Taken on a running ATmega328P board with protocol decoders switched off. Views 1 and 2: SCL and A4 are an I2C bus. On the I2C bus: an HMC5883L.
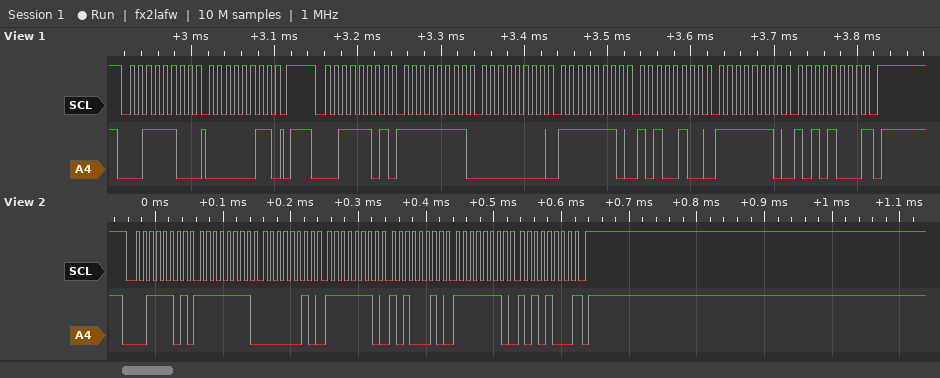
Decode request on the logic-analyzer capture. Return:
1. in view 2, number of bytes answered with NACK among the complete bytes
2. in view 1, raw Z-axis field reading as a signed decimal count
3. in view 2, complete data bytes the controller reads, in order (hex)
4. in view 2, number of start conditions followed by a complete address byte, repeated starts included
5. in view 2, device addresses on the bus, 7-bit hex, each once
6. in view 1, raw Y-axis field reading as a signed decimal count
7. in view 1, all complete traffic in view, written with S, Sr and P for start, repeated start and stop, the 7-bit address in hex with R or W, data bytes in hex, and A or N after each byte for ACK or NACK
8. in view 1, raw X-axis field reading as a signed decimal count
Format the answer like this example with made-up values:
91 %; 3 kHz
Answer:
1; -348; FF 02 FE A2 FE A8; 1; 0x1E; -344; S 1EW A 03 A P S 1ER A FF A 00 A FE A A4 A FE A A8 N P; -256
